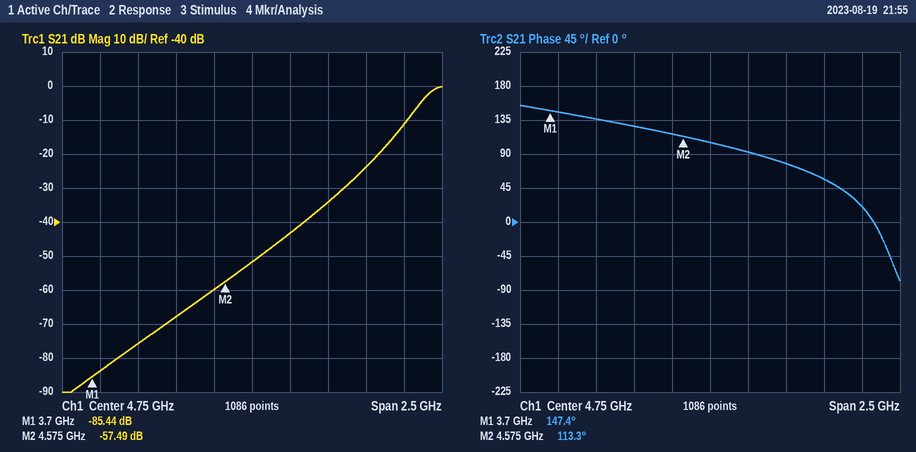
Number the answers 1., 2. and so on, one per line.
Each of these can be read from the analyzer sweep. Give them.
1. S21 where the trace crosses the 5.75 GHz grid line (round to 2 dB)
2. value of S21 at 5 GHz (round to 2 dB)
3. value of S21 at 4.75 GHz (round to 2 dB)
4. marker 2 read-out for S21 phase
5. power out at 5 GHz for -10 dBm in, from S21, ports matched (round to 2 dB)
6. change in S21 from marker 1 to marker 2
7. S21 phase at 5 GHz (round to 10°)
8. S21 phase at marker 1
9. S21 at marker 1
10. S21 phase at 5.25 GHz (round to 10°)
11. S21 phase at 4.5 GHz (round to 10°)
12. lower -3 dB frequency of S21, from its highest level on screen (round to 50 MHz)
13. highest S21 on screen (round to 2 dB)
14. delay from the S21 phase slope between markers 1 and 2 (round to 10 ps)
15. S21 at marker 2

1. -12 dB
2. -44 dB
3. -52 dB
4. 113.3°
5. -54 dBm
6. 27.95 dB
7. 90°
8. 147.4°
9. -85.44 dB
10. 80°
11. 120°
12. 5.90 GHz
13. 0 dB
14. 110 ps
15. -57.49 dB
